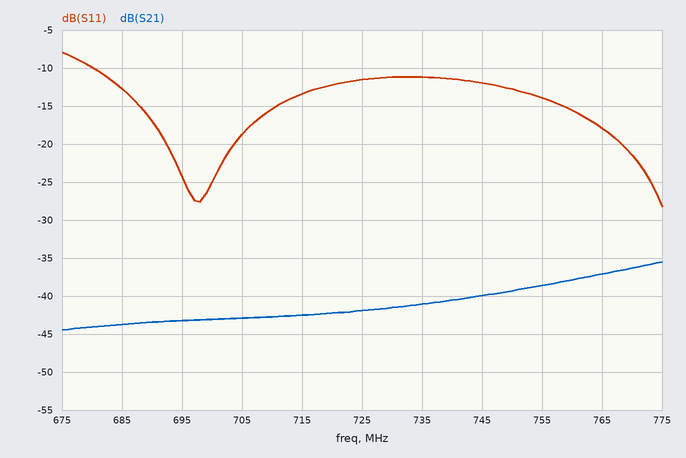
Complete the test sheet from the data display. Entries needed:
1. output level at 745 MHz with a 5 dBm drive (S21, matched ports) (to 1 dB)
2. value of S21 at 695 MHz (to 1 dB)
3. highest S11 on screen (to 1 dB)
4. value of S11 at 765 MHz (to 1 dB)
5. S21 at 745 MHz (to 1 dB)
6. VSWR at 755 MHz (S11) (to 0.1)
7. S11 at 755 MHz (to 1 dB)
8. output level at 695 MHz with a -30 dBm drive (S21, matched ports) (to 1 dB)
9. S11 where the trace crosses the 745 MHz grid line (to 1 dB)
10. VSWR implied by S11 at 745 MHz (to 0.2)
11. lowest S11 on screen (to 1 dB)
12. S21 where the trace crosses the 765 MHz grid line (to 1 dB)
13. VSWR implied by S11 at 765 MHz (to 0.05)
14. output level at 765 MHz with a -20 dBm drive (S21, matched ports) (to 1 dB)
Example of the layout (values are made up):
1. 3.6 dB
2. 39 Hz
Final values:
1. -35 dBm
2. -43 dB
3. -8 dB
4. -18 dB
5. -40 dB
6. 1.5
7. -14 dB
8. -73 dBm
9. -12 dB
10. 1.6
11. -28 dB
12. -37 dB
13. 1.30
14. -57 dBm
